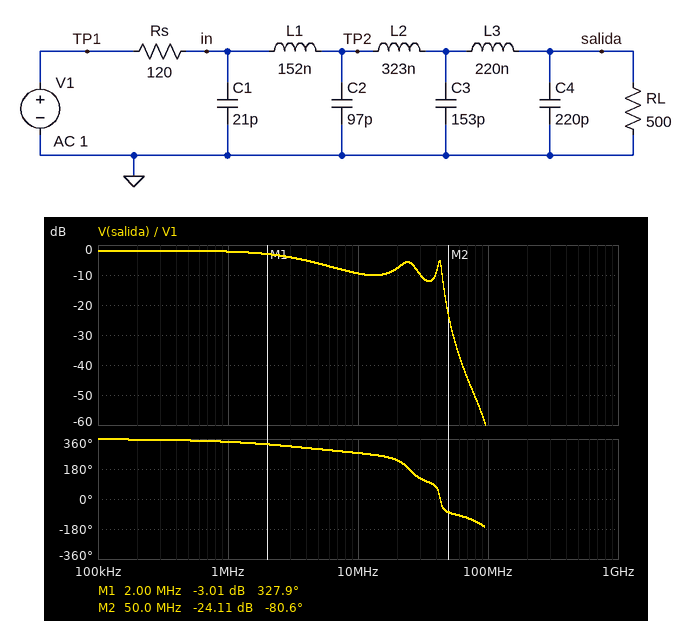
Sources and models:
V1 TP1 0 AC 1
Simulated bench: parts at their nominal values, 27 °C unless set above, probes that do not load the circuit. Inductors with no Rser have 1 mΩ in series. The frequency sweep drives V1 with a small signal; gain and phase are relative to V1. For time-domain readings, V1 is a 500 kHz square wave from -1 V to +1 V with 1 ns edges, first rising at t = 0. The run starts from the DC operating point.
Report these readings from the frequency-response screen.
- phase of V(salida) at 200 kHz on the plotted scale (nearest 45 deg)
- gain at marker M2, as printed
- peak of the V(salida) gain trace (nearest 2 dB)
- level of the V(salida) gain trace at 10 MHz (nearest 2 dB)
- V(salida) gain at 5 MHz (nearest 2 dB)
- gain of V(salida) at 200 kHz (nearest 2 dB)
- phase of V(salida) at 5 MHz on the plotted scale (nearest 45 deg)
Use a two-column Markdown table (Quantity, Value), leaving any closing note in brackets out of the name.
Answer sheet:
| Quantity | Value |
|---|---|
| phase of V(salida) at 200 kHz on the plotted scale | 360 deg |
| gain at marker M2, as printed | -24.11 dB |
| peak of the V(salida) gain trace | -2 dB |
| level of the V(salida) gain trace at 10 MHz | -10 dB |
| V(salida) gain at 5 MHz | -6 dB |
| gain of V(salida) at 200 kHz | -2 dB |
| phase of V(salida) at 5 MHz on the plotted scale | 315 deg |
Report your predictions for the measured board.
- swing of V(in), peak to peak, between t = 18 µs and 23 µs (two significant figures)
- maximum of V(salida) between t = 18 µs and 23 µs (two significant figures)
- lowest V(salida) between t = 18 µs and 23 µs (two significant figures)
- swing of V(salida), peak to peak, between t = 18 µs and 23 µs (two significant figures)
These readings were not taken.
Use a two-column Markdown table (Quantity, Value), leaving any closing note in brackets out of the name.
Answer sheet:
| Quantity | Value |
|---|---|
| swing of V(in), peak to peak, between t = 18 µs and 23 µs | 1.6 V |
| maximum of V(salida) between t = 18 µs and 23 µs | 810 mV |
| lowest V(salida) between t = 18 µs and 23 µs | -810 mV |
| swing of V(salida), peak to peak, between t = 18 µs and 23 µs | 1.6 V |
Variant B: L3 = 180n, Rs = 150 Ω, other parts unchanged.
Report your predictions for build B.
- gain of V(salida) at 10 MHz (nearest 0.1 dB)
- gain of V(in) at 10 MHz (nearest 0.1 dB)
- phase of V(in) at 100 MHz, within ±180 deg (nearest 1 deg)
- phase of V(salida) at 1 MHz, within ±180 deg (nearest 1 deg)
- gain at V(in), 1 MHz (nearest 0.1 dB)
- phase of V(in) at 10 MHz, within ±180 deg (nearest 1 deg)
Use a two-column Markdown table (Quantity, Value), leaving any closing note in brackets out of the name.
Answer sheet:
| Quantity | Value |
|---|---|
| gain of V(salida) at 10 MHz | -11.5 dB |
| gain of V(in) at 10 MHz | -26.4 dB |
| phase of V(in) at 100 MHz, within ±180 deg | -3 deg |
| phase of V(salida) at 1 MHz, within ±180 deg | -20 deg |
| gain at V(in), 1 MHz | -2.8 dB |
| phase of V(in) at 10 MHz, within ±180 deg | -61 deg |
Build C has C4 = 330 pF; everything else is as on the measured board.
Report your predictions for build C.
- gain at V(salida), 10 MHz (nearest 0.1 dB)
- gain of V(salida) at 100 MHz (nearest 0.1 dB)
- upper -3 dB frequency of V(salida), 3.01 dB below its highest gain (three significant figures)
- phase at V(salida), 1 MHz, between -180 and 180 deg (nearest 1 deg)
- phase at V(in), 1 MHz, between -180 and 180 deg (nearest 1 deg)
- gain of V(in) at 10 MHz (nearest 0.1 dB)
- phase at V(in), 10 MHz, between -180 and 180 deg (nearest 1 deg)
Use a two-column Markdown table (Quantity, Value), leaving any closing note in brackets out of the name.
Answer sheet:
| Quantity | Value |
|---|---|
| gain at V(salida), 10 MHz | -10.8 dB |
| gain of V(salida) at 100 MHz | -66.2 dB |
| upper -3 dB frequency of V(salida), 3.01 dB below its highest gain | 2.99 MHz |
| phase at V(salida), 1 MHz, between -180 and 180 deg | -21 deg |
| phase at V(in), 1 MHz, between -180 and 180 deg | -20 deg |
| gain of V(in) at 10 MHz | -27.8 dB |
| phase at V(in), 10 MHz, between -180 and 180 deg | 58 deg |
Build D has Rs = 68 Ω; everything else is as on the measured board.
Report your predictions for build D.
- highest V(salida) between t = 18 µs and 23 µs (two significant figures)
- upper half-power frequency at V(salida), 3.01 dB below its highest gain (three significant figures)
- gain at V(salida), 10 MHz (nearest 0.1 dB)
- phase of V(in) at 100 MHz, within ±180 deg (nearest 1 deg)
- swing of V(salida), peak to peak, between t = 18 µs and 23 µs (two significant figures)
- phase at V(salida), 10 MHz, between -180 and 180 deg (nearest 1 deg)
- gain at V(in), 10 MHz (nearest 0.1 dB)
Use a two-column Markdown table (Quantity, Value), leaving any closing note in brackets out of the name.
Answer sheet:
| Quantity | Value |
|---|---|
| highest V(salida) between t = 18 µs and 23 µs | 890 mV |
| upper half-power frequency at V(salida), 3.01 dB below its highest gain | 8.19 MHz |
| gain at V(salida), 10 MHz | -4.7 dB |
| phase of V(in) at 100 MHz, within ±180 deg | -1 deg |
| swing of V(salida), peak to peak, between t = 18 µs and 23 µs | 1.8 V |
| phase at V(salida), 10 MHz, between -180 and 180 deg | -82 deg |
| gain at V(in), 10 MHz | -20.6 dB |
